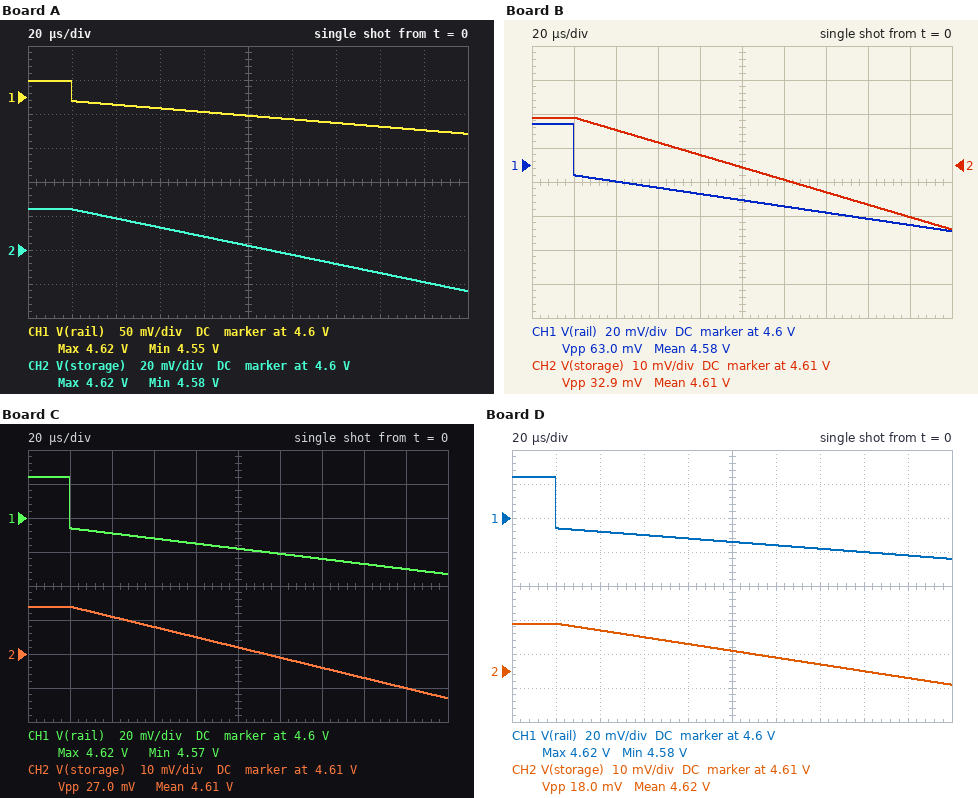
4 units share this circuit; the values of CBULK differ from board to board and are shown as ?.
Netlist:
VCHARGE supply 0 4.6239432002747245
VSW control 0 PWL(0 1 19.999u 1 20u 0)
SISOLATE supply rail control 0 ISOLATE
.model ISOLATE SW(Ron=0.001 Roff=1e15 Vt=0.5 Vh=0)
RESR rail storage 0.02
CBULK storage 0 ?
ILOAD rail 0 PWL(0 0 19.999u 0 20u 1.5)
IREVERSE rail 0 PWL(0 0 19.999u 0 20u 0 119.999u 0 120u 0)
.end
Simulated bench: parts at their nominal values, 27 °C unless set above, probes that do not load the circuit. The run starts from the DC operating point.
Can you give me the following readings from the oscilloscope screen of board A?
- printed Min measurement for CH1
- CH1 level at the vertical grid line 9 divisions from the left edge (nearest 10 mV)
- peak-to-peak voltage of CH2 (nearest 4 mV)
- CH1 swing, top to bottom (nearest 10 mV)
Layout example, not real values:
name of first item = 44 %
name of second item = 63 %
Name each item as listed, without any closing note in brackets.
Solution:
printed Min measurement for CH1 = 4.55 V
CH1 level at the vertical grid line 9 divisions from the left edge = 4.55 V
peak-to-peak voltage of CH2 = 48 mV
CH1 swing, top to bottom = 80 mV
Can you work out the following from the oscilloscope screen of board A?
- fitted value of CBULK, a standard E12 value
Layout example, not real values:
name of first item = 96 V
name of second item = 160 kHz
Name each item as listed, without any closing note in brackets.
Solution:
fitted value of CBULK, a standard E12 value = 5.6 mF
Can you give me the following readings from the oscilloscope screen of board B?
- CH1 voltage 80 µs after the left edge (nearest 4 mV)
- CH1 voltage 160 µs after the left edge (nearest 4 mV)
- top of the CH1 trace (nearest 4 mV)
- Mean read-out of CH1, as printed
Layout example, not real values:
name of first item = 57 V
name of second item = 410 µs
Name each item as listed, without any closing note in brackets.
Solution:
CH1 voltage 80 µs after the left edge = 4.584 V
CH1 voltage 160 µs after the left edge = 4.568 V
top of the CH1 trace = 4.624 V
Mean read-out of CH1, as printed = 4.58 V
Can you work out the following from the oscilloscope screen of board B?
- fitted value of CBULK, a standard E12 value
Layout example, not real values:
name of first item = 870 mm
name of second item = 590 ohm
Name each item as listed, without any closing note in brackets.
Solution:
fitted value of CBULK, a standard E12 value = 8.2 mF
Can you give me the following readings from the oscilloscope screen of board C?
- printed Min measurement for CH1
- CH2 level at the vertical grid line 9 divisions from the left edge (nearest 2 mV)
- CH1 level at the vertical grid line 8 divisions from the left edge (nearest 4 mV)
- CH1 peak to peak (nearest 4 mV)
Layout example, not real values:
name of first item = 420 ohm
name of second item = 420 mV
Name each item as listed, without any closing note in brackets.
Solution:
printed Min measurement for CH1 = 4.57 V
CH2 level at the vertical grid line 9 divisions from the left edge = 4.600 V
CH1 level at the vertical grid line 8 divisions from the left edge = 4.572 V
CH1 peak to peak = 56 mV
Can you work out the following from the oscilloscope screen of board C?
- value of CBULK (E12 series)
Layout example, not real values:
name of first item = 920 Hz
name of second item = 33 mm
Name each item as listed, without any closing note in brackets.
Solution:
value of CBULK = 10 mF
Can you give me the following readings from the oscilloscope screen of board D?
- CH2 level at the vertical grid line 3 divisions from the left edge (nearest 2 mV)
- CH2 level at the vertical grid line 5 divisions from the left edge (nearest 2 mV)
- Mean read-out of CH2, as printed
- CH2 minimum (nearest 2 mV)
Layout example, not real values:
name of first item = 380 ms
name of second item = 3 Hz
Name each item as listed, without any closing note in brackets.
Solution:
CH2 level at the vertical grid line 3 divisions from the left edge = 4.620 V
CH2 level at the vertical grid line 5 divisions from the left edge = 4.616 V
Mean read-out of CH2, as printed = 4.62 V
CH2 minimum = 4.606 V
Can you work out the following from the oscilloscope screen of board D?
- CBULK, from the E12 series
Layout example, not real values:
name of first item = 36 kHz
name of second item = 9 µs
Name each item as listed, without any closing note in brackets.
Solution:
CBULK, from the E12 series = 15 mF
